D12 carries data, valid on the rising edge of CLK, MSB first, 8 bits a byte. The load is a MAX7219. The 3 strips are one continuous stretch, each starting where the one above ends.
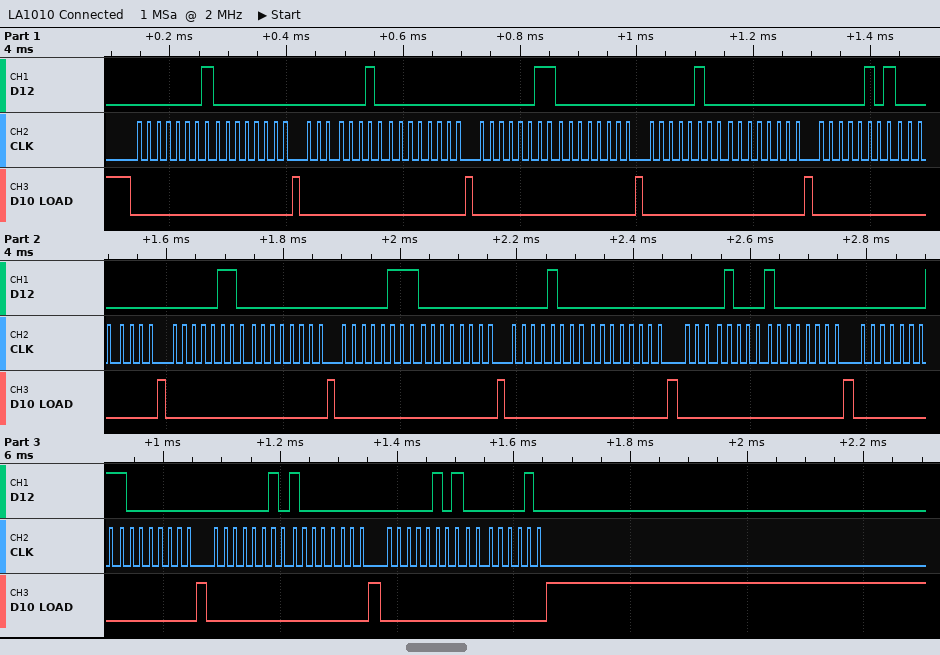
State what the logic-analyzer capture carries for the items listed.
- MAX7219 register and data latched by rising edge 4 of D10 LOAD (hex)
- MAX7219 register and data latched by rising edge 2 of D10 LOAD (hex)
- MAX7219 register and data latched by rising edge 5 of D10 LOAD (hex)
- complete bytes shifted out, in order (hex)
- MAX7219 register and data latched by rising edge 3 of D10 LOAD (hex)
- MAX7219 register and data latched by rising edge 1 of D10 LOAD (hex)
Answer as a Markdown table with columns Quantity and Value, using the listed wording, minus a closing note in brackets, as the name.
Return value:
| Quantity | Value |
|---|---|
| MAX7219 register and data latched by rising edge 4 of D10 LOAD | register 0x4, data 0x00 |
| MAX7219 register and data latched by rising edge 2 of D10 LOAD | register 0x2, data 0x00 |
| MAX7219 register and data latched by rising edge 5 of D10 LOAD | register 0x5, data 0x00 |
| complete bytes shifted out, in order | 0x01 0x00 0x02 0x00 0x03 0x00 0x04 0x00 0x05 0x00 0x06 0x00 0x07 0x00 0x08 0x00 0x08 0x80 0x01 0x80 0x02 0x80 0x05 0x02 |
| MAX7219 register and data latched by rising edge 3 of D10 LOAD | register 0x3, data 0x00 |
| MAX7219 register and data latched by rising edge 1 of D10 LOAD | register 0x1, data 0x00 |
